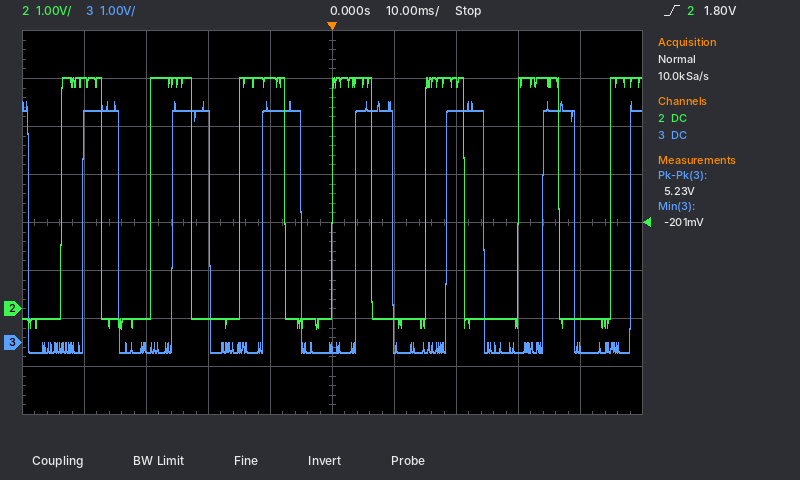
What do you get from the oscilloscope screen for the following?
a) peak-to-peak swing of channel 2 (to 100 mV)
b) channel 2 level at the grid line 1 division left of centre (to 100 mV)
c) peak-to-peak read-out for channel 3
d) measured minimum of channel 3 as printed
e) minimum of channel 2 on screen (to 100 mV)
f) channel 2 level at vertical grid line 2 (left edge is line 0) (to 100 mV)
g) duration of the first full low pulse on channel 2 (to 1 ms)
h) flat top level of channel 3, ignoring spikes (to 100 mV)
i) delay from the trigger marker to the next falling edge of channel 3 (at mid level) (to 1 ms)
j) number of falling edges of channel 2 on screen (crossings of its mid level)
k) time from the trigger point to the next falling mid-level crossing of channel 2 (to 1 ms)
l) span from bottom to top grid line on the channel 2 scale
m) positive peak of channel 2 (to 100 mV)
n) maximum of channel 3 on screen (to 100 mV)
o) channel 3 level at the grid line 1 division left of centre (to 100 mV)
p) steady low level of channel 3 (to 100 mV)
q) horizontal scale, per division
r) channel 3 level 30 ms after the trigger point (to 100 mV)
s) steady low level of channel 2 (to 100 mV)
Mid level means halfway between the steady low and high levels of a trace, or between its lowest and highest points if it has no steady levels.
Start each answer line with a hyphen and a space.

- 5.2 V
- 4.8 V
- 5.23 V
- -201 mV
- -400 mV
- -200 mV
- 8 ms
- 4.8 V
- 10 ms
- 6
- 6 ms
- 8 V
- 4.8 V
- 5.0 V
- 4.9 V
- -200 mV
- 10 ms
- -200 mV
- -200 mV
